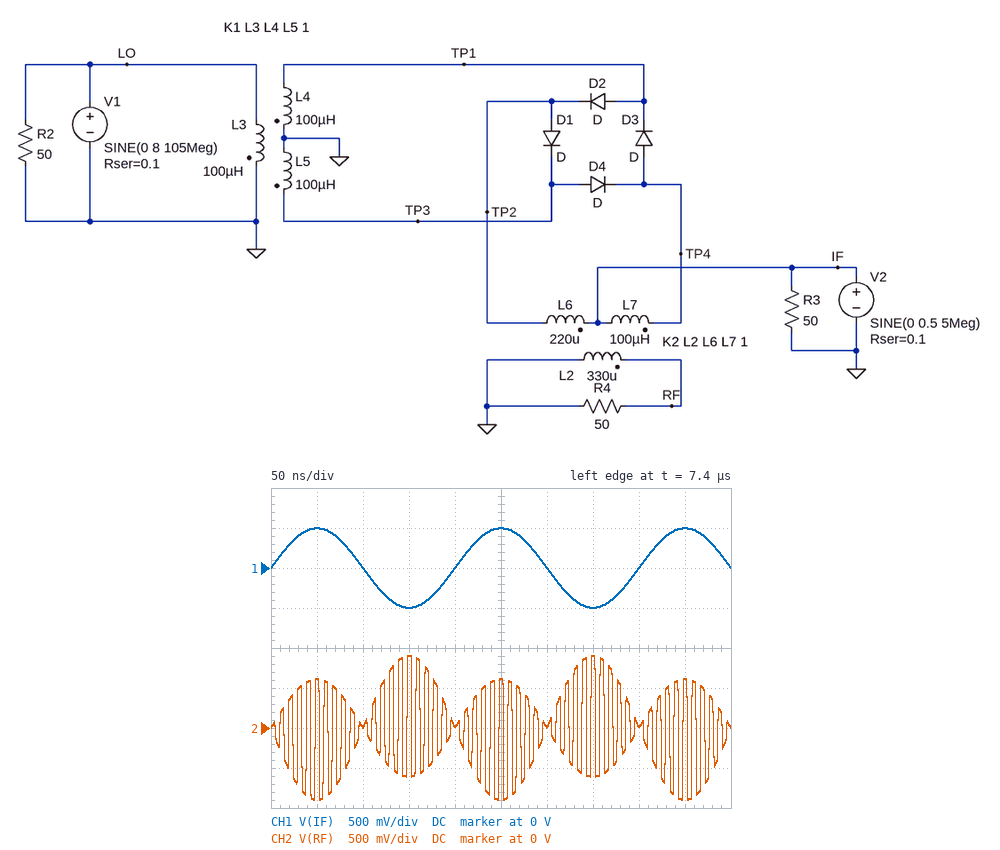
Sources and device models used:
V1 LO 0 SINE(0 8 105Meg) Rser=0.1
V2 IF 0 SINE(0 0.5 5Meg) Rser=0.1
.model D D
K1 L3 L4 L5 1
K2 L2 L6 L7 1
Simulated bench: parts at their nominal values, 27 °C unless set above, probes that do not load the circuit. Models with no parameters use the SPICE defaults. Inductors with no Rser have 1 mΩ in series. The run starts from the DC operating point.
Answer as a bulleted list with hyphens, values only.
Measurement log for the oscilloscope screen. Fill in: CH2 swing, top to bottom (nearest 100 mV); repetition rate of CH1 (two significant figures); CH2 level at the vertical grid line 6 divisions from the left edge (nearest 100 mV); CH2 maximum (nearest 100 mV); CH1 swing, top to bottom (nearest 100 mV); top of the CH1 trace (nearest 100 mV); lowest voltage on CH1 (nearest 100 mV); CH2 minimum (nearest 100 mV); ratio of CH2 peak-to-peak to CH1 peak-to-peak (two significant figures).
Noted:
- 1.8 V
- 5.0 MHz
- 0 V
- 900 mV
- 1.0 V
- 500 mV
- -500 mV
- -900 mV
- 1.8
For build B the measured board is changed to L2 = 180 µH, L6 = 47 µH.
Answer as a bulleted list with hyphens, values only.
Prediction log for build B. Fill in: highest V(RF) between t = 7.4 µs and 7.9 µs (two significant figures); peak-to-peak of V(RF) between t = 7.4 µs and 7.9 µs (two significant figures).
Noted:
- 970 mV
- 1.9 V
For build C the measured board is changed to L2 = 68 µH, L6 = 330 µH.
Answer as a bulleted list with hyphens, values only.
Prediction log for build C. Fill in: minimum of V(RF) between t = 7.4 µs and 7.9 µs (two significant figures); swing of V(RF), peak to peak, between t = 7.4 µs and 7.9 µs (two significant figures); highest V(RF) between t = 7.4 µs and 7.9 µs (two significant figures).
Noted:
- -410 mV
- 820 mV
- 410 mV
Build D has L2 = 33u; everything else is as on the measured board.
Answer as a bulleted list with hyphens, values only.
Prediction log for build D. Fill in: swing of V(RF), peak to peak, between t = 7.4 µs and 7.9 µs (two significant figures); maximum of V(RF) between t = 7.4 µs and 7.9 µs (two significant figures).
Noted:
- 570 mV
- 290 mV
